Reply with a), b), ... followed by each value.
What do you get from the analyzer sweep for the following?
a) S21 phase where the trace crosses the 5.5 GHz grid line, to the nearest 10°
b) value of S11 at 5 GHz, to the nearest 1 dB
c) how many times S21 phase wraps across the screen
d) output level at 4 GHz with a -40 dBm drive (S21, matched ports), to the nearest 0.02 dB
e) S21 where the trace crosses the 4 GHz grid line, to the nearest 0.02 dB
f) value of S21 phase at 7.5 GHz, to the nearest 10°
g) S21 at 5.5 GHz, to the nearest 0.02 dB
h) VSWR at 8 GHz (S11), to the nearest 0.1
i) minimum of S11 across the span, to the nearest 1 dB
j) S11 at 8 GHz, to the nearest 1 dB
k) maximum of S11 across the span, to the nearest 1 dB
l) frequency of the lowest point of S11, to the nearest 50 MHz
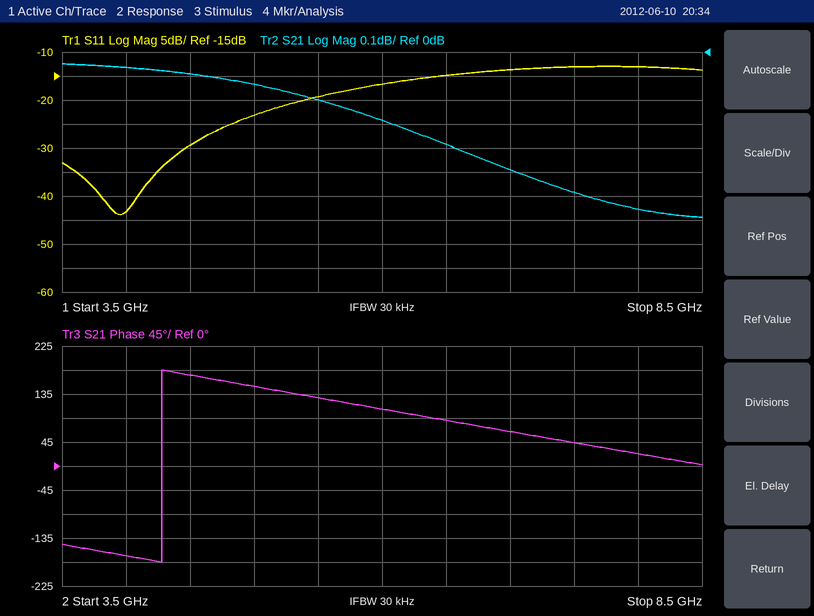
a) 130°
b) -23 dB
c) 1
d) -40.06 dBm
e) -0.06 dB
f) 40°
g) -0.20 dB
h) 1.6
i) -44 dB
j) -13 dB
k) -13 dB
l) 3.95 GHz
